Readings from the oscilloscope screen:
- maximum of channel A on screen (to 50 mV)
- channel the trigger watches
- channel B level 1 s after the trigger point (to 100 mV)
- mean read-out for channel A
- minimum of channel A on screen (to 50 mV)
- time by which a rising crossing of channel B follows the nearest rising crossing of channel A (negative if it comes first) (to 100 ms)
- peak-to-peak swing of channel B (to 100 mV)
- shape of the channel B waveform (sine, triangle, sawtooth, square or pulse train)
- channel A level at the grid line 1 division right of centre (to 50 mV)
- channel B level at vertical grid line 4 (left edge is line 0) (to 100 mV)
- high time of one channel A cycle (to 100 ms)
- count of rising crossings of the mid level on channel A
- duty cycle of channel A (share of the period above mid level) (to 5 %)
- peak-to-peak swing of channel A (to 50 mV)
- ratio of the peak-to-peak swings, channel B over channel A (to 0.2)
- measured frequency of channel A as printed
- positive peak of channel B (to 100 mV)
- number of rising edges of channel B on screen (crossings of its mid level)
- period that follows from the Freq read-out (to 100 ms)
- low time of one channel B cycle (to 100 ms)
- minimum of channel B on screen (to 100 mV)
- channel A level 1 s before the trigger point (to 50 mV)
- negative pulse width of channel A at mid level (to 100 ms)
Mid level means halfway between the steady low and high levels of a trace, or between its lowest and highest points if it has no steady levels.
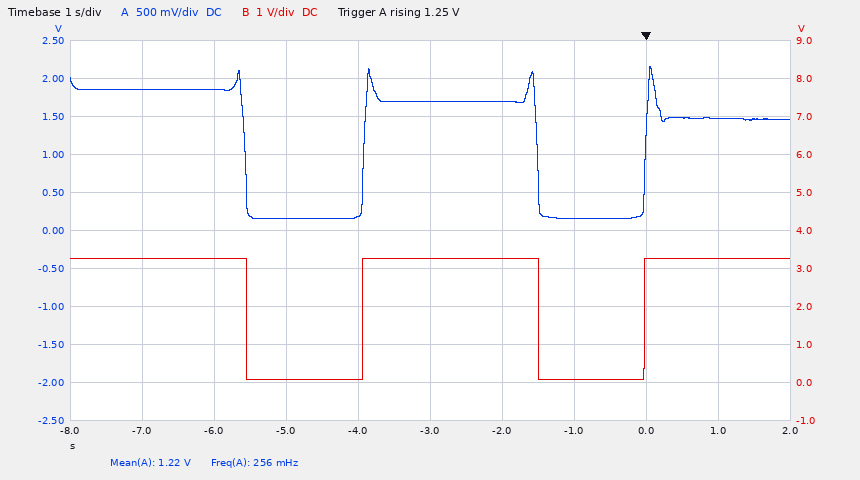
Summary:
2.15 V
channel A
3.3 V
1.22 V
150 mV
0.0 s
3.2 V
pulse train
1.70 V
100 mV
2.4 s
2
60 %
2.00 V
1.6
256 mHz
3.3 V
2
3.9 s
1.5 s
100 mV
150 mV
1.5 s
